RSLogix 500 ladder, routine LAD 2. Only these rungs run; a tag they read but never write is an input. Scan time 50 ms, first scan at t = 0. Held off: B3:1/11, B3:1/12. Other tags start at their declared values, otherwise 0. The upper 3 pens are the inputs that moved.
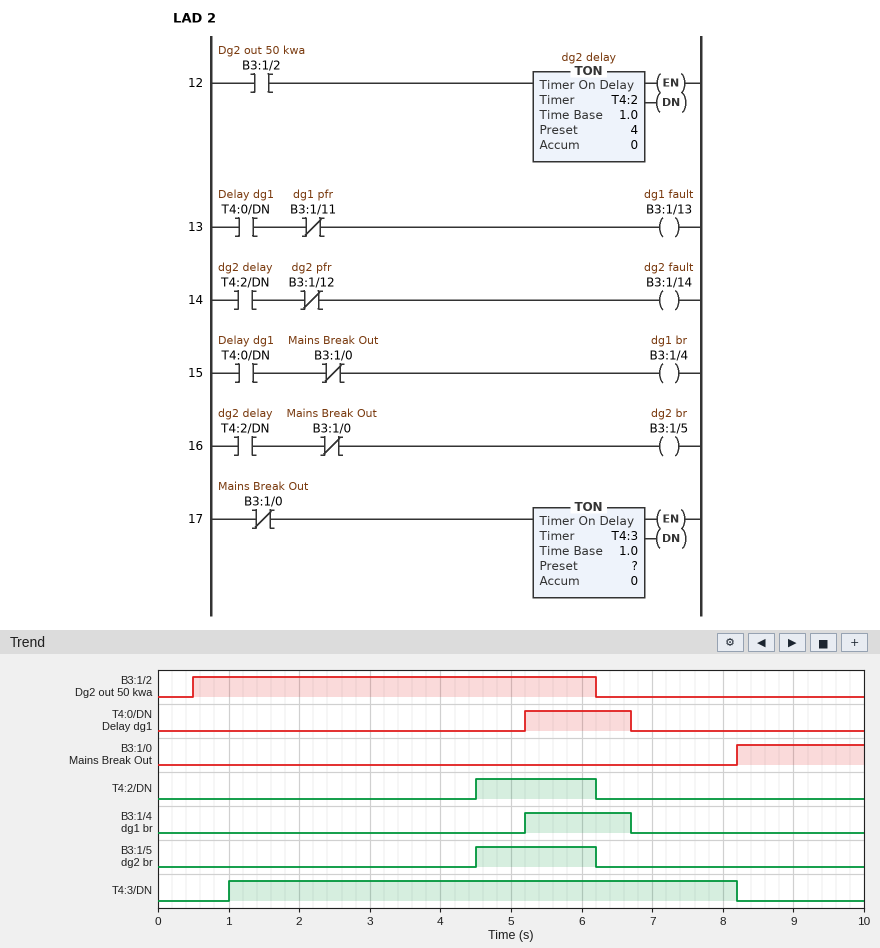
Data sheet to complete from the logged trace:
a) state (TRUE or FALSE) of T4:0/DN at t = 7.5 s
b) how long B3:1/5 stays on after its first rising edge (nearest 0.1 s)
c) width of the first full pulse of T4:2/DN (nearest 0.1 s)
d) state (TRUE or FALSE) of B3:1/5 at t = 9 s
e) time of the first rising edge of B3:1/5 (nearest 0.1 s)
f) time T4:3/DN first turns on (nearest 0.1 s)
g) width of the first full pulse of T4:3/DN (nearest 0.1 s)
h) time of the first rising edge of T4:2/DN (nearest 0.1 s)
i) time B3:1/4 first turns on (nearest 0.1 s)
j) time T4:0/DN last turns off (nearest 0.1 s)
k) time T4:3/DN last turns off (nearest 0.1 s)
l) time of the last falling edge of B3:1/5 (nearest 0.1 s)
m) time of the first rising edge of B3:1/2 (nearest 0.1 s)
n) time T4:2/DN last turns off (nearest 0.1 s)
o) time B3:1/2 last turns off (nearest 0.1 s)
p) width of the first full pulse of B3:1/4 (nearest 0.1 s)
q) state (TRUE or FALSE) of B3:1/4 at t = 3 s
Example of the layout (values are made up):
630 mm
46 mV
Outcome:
FALSE
1.7 s
1.7 s
FALSE
4.5 s
1.0 s
7.2 s
4.5 s
5.2 s
6.7 s
8.2 s
6.2 s
0.5 s
6.2 s
6.2 s
1.5 s
FALSE
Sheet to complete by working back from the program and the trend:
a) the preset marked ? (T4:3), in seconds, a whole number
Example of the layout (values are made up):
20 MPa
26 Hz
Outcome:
1 s
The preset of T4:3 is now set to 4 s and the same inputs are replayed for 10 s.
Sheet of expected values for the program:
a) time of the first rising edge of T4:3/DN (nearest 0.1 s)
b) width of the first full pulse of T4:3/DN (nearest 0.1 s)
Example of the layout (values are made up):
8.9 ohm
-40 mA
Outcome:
4.0 s
4.2 s
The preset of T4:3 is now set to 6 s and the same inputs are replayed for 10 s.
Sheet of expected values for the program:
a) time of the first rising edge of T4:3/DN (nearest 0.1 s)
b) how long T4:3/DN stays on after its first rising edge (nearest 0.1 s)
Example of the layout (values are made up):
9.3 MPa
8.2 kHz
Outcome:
6.0 s
2.2 s
